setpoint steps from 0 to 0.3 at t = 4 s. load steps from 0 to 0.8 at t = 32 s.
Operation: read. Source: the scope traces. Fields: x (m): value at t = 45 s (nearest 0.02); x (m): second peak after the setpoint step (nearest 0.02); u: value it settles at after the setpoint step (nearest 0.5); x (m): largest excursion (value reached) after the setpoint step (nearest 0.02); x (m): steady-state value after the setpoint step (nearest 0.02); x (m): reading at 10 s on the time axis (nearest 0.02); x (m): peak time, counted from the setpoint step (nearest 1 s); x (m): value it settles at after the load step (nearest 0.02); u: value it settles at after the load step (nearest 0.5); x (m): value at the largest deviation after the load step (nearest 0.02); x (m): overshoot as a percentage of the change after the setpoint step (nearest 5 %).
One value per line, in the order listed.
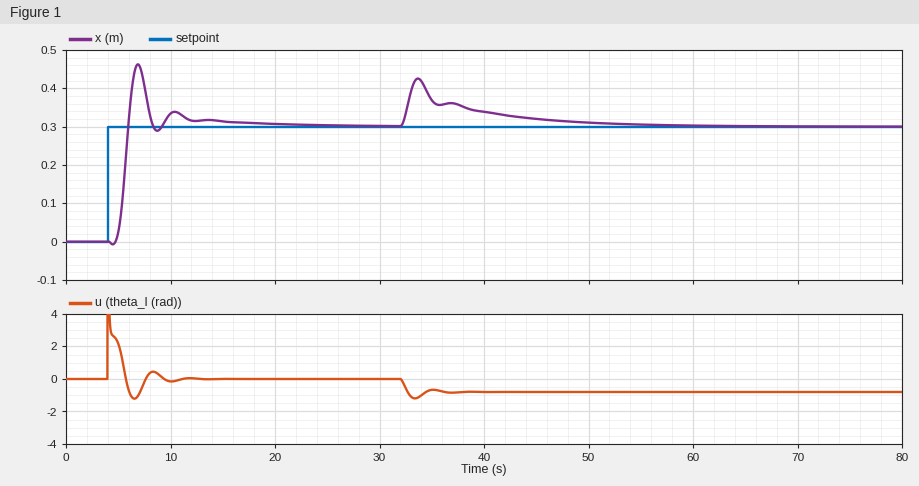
0.32
0.34
0.0
0.46
0.30
0.34
3 s
0.30
-1.0
0.42
55 %
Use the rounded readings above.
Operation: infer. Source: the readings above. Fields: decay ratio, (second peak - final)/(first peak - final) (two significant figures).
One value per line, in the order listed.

0.25
